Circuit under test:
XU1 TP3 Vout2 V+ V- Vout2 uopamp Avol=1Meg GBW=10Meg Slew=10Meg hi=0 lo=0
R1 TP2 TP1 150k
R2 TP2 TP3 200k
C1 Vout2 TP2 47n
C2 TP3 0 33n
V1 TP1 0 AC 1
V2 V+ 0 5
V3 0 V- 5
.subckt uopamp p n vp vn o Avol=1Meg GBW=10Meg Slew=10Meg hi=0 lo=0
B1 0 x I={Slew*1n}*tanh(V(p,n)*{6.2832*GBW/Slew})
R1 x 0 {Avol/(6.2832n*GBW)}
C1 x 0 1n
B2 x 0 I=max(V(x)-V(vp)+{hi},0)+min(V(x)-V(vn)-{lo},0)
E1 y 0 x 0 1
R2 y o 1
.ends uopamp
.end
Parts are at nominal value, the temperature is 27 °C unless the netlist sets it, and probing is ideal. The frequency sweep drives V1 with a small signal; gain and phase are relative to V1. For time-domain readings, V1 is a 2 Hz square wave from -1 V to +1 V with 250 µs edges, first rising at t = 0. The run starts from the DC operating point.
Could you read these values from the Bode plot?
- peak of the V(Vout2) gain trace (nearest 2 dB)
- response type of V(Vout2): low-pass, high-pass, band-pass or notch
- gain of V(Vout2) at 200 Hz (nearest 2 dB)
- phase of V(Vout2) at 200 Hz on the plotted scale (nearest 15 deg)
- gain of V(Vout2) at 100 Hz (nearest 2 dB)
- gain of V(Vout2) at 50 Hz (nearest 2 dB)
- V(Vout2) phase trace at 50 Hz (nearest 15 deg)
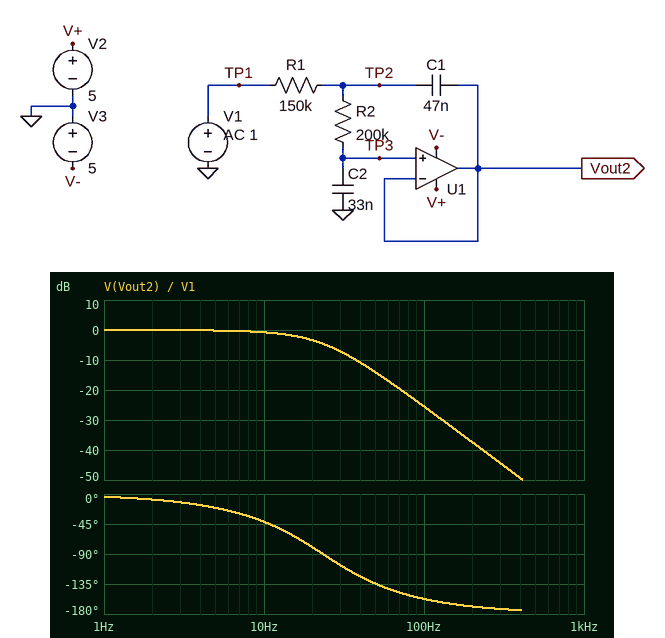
0 dB
low-pass
-38 dB
-165 deg
-26 dB
-14 dB
-135 deg
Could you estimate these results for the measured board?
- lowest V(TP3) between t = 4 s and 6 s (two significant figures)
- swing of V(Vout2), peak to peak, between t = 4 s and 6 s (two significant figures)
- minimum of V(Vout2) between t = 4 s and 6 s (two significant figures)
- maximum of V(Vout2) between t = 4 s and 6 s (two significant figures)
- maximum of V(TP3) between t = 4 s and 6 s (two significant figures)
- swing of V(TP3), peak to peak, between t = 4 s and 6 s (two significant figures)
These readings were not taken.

-1.0 V
2.0 V
-1.0 V
1.0 V
1.0 V
2.0 V
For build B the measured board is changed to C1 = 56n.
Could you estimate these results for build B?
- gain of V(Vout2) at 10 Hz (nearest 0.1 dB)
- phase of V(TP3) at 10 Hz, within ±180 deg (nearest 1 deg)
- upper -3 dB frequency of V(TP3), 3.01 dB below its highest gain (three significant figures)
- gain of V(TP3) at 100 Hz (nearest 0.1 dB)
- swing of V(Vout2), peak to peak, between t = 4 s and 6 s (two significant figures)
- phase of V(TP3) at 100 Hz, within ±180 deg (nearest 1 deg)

-0.6 dB
-43 deg
19.3 Hz
-26.9 dB
2.1 V
-161 deg
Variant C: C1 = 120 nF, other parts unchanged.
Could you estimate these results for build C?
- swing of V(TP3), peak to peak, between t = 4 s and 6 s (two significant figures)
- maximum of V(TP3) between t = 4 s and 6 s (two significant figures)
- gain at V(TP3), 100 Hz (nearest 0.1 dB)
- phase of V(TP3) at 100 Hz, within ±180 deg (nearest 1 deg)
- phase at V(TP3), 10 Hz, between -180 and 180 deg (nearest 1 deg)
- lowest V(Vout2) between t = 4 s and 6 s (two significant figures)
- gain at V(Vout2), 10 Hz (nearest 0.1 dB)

2.6 V
1.3 V
-33.3 dB
-171 deg
-54 deg
-1.3 V
0.9 dB
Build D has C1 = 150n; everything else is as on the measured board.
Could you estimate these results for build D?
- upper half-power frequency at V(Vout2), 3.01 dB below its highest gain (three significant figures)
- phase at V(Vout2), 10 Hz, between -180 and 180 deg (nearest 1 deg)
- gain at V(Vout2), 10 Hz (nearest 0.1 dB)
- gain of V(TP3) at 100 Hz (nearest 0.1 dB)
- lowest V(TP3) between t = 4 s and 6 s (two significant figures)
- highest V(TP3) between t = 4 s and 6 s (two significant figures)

15.4 Hz
-60 deg
1.6 dB
-35.3 dB
-1.4 V
1.4 V
